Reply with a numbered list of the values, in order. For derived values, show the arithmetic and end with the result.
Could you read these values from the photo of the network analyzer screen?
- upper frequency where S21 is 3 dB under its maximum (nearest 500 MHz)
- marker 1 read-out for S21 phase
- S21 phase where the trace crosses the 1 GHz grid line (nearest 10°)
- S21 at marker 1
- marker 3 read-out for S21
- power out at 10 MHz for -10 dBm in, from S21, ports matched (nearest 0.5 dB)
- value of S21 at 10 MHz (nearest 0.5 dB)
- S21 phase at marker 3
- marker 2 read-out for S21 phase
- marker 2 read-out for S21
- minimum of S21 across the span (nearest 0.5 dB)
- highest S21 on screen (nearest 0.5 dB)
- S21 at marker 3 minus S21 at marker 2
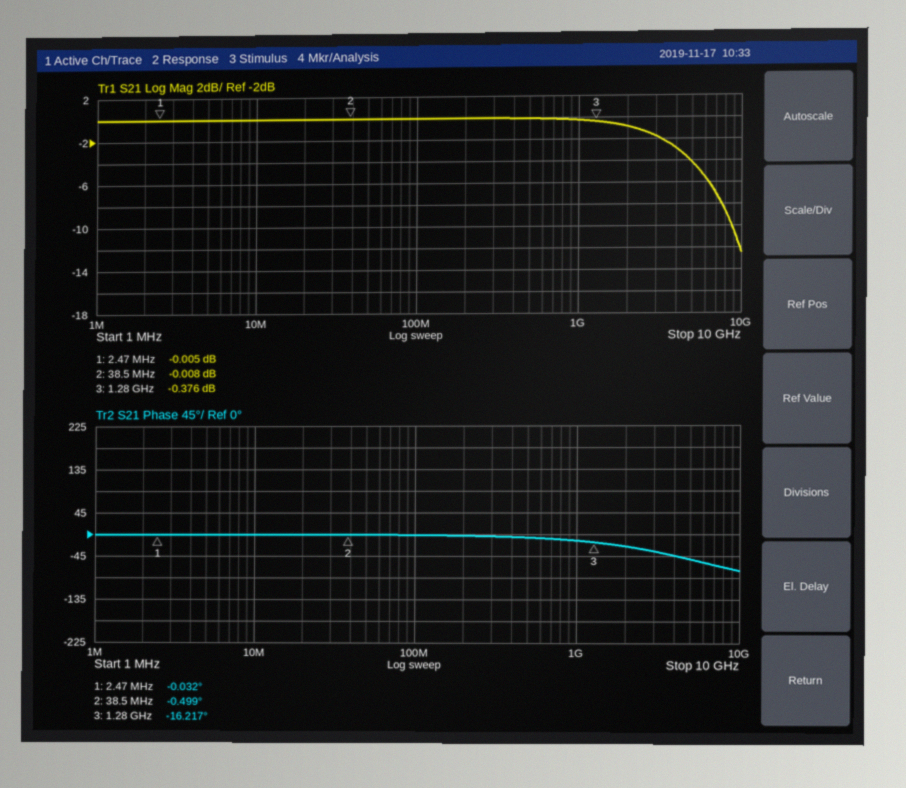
1. 4.0 GHz
2. -0.032°
3. -10°
4. -0.005 dB
5. -0.376 dB
6. -10 dBm + (0.0 dB) = -10.0 dBm
7. 0.0 dB
8. -16.217°
9. -0.499°
10. -0.008 dB
11. -12.5 dB
12. 0.0 dB
13. -0.376 − (-0.008) = -0.368 dB
